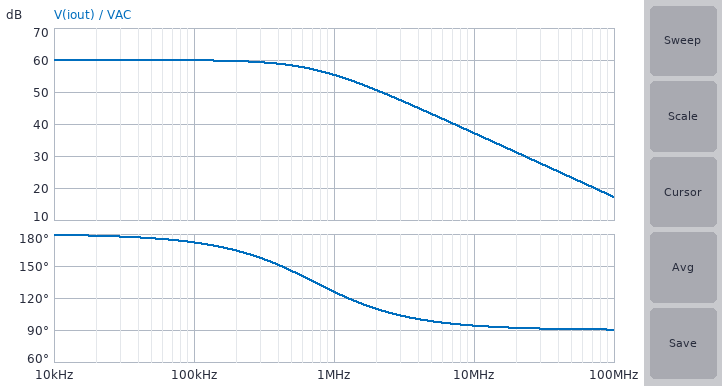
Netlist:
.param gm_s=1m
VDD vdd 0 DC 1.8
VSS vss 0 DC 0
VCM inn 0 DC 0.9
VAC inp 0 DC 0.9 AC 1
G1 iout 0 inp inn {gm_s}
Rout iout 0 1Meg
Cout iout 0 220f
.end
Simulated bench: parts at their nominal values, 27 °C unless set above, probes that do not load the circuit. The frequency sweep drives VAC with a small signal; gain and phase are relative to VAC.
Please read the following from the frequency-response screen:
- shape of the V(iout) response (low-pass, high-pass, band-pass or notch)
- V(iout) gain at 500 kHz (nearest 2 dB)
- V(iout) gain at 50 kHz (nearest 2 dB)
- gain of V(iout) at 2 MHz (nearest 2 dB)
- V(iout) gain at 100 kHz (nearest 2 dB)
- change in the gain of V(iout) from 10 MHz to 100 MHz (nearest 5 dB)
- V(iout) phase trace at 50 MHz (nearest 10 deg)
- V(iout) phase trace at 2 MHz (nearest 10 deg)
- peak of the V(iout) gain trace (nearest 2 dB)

low-pass
58 dB
60 dB
50 dB
60 dB
-20 dB
90 deg
110 deg
60 dB
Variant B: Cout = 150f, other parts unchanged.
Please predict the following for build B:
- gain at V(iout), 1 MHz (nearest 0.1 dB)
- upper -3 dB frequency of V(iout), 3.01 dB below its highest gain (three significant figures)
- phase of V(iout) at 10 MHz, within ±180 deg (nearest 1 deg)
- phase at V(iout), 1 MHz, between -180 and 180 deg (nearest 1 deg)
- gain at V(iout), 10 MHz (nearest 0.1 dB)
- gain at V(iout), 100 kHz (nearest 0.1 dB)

57.2 dB
1.06 MHz
96 deg
137 deg
40.5 dB
60.0 dB
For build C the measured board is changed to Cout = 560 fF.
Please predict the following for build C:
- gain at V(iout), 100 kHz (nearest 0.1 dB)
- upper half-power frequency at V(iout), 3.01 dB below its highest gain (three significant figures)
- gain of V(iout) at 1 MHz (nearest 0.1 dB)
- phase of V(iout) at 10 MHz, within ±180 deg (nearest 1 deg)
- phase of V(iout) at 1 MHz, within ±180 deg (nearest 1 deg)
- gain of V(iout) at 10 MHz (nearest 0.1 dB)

59.5 dB
284 kHz
48.7 dB
92 deg
106 deg
29.1 dB
